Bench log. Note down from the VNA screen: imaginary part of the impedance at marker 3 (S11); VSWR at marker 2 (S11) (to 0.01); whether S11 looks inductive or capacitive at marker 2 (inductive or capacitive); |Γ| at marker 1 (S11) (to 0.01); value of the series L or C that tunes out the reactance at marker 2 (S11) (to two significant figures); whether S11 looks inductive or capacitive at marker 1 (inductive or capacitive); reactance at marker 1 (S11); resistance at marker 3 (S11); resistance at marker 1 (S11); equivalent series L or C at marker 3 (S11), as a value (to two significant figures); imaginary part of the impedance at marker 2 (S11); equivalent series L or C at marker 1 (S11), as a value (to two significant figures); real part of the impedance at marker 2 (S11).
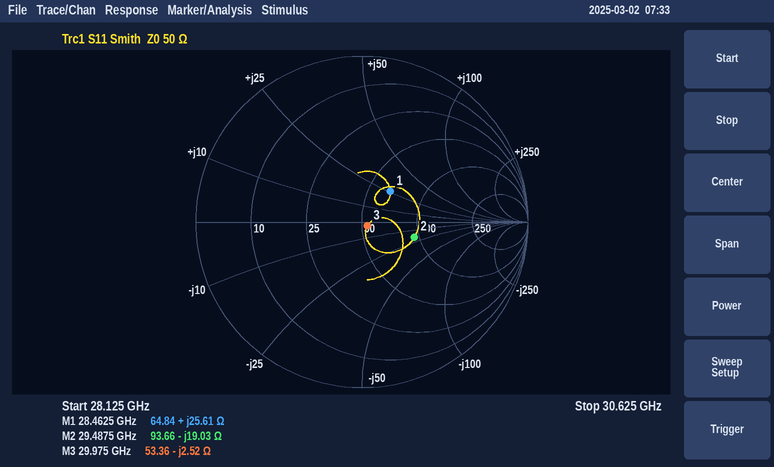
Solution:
-2.52 Ω
1.98
capacitive
0.25
100 pH
inductive
+25.61 Ω
53.36 Ω
64.84 Ω
2.1 pF
-19.03 Ω
140 pH
93.66 Ω
